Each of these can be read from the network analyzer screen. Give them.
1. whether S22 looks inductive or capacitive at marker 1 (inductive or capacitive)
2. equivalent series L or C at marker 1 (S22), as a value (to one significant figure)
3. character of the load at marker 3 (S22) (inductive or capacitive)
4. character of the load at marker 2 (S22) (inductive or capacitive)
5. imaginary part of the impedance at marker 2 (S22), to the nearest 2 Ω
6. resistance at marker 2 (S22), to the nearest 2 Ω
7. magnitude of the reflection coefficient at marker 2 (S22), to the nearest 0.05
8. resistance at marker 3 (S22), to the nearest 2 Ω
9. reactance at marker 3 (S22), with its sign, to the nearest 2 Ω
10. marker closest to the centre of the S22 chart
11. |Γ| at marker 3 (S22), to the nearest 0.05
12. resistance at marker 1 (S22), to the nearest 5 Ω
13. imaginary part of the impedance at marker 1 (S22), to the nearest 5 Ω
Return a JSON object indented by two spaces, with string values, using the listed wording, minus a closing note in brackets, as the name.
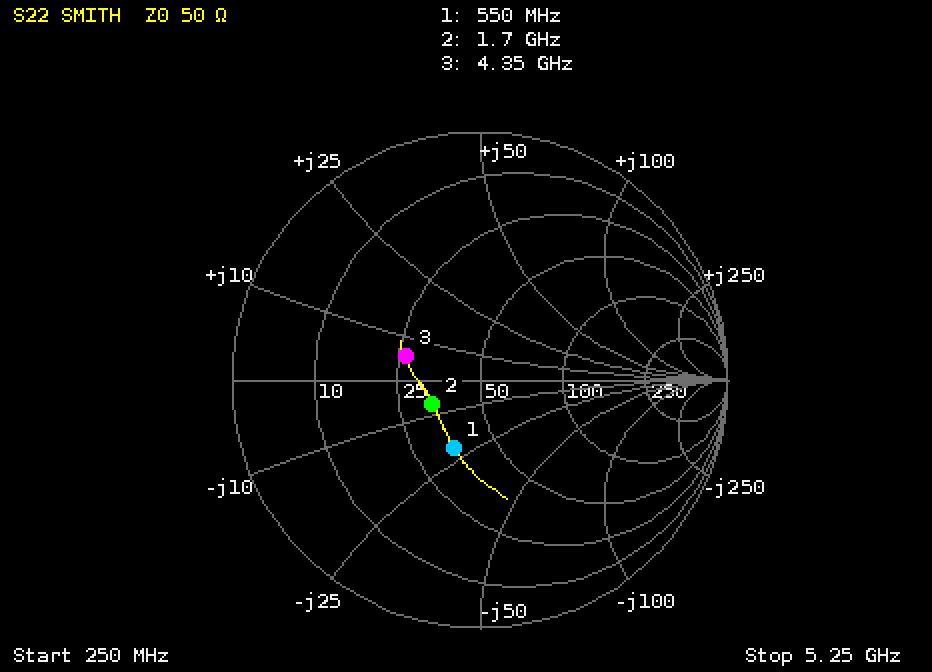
{
  "whether S22 looks inductive or capacitive at marker 1": "capacitive",
  "equivalent series L or C at marker 1 (S22), as a value": "10 pF",
  "character of the load at marker 3 (S22)": "inductive",
  "character of the load at marker 2 (S22)": "capacitive",
  "imaginary part of the impedance at marker 2 (S22), to the nearest 2 Ω": "-6 Ω",
  "resistance at marker 2 (S22), to the nearest 2 Ω": "34 Ω",
  "magnitude of the reflection coefficient at marker 2 (S22), to the nearest 0.05": "0.20",
  "resistance at marker 3 (S22), to the nearest 2 Ω": "26 Ω",
  "reactance at marker 3 (S22), with its sign, to the nearest 2 Ω": "+6 Ω",
  "marker closest to the centre of the S22 chart": "marker 2",
  "|Γ| at marker 3 (S22), to the nearest 0.05": "0.30",
  "resistance at marker 1 (S22), to the nearest 5 Ω": "35 Ω",
  "imaginary part of the impedance at marker 1 (S22), to the nearest 5 Ω": "-20 Ω"
}
